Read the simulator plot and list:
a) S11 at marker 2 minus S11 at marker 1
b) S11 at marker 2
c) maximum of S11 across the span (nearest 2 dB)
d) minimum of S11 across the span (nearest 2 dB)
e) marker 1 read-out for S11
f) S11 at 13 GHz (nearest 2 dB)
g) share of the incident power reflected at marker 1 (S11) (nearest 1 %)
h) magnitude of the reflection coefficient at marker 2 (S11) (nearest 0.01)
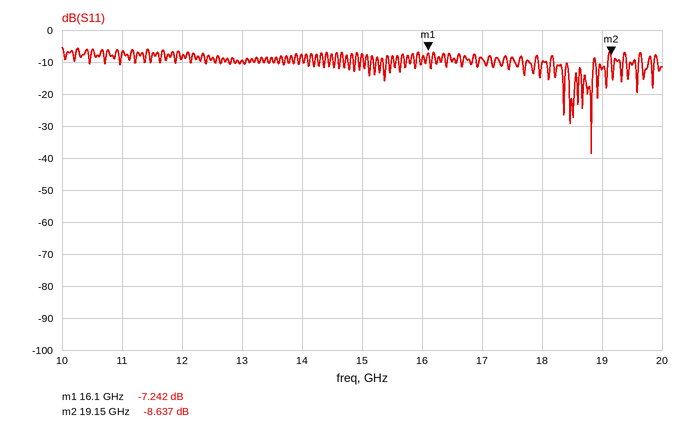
-1.395 dB
-8.637 dB
-6 dB
-38 dB
-7.242 dB
-10 dB
19 %
0.37
